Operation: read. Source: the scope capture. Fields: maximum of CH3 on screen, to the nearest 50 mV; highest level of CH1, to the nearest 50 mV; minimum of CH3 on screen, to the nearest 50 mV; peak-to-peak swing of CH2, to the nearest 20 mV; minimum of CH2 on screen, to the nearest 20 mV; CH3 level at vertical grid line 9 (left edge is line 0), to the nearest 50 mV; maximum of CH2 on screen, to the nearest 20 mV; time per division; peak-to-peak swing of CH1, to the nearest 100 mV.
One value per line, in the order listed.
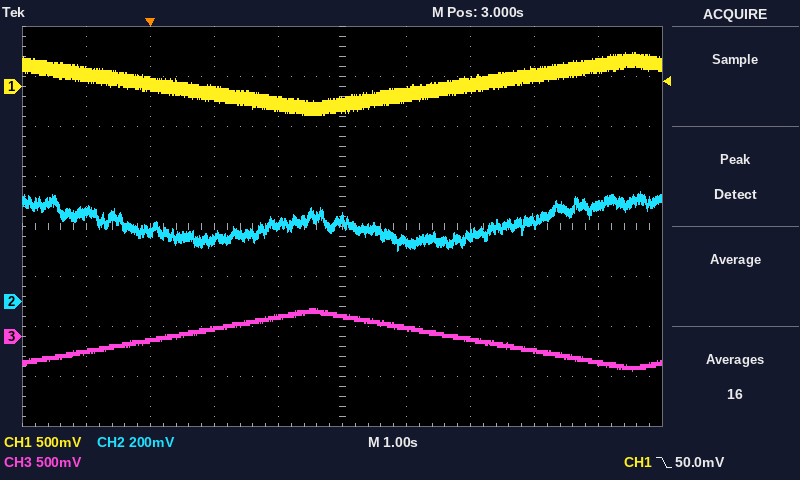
300 mV
350 mV
-350 mV
240 mV
200 mV
-250 mV
440 mV
1 s
600 mV
